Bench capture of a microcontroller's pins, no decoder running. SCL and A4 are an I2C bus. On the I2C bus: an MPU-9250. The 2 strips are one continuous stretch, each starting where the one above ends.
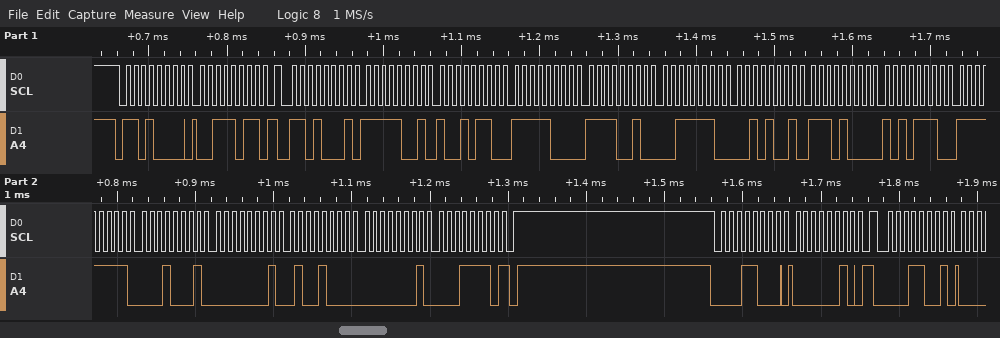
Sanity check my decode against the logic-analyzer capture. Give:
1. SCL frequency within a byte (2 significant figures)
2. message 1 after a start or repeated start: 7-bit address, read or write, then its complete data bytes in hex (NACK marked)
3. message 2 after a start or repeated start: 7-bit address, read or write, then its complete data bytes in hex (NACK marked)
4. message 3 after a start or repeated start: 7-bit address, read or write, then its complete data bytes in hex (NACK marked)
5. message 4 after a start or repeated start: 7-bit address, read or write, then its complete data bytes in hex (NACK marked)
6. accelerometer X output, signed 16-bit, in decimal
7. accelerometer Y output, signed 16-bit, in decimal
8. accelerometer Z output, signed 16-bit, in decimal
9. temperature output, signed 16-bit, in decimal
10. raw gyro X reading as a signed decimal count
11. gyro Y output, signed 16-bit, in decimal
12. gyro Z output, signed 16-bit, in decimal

100 kHz
0x68 write: 3B
0x68 read: F9 96 F8 F2 3E 29 E8 AE FF 11 01 48 01 1E NACK
0x0C write: 02
0x0C read
-1642
-1806
15913
-5970
-239
328
286
